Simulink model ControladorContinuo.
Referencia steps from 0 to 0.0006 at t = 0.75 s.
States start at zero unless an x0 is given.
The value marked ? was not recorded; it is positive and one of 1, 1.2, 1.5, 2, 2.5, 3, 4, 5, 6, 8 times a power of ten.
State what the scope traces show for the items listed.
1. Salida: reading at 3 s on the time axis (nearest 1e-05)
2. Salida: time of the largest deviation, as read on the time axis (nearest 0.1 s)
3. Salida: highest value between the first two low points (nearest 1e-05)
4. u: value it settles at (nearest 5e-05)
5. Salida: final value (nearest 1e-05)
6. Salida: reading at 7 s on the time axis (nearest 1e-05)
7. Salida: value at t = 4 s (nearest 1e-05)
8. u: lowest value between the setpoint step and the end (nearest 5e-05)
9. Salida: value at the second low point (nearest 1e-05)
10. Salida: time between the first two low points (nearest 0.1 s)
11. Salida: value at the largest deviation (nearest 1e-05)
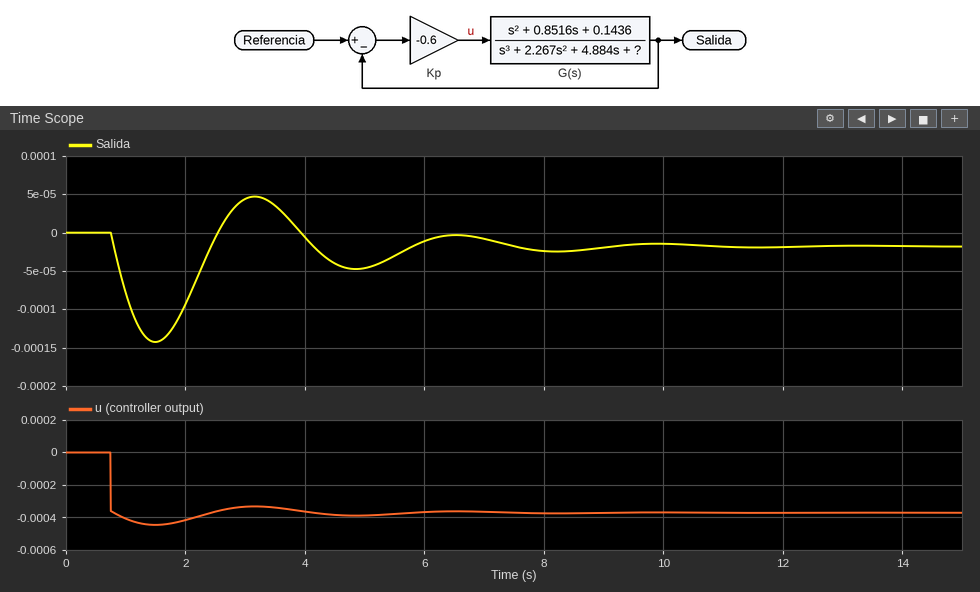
0.00004
1.5 s
0.00005
-0.00035
-0.00002
-0.00001
-0.00001
-0.00045
-0.00005
3.4 s
-0.00014
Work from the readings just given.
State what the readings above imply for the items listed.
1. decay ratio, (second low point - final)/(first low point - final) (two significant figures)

0.25
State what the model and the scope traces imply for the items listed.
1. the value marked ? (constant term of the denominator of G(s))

3
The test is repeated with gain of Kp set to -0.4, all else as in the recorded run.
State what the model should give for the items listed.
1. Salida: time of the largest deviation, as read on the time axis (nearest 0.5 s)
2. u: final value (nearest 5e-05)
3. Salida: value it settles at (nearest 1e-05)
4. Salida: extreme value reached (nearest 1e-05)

1.5 s
-0.00025
-0.00001
-0.00009
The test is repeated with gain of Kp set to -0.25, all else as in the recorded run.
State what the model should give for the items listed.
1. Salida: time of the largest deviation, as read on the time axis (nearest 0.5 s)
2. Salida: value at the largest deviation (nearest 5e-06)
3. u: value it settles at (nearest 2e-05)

1.5 s
-0.000055
-0.00016
